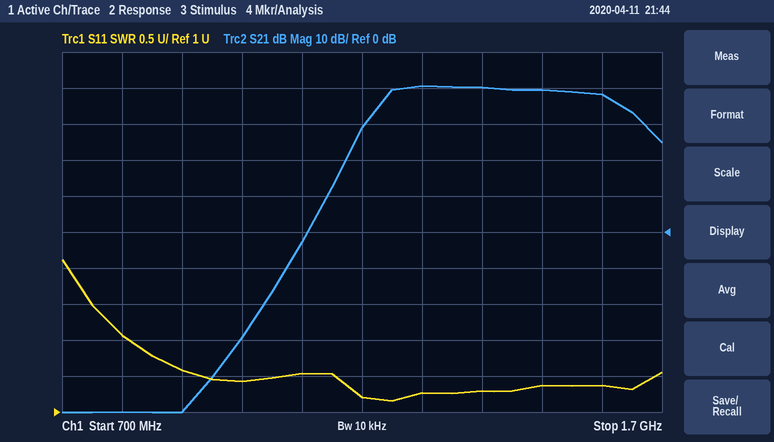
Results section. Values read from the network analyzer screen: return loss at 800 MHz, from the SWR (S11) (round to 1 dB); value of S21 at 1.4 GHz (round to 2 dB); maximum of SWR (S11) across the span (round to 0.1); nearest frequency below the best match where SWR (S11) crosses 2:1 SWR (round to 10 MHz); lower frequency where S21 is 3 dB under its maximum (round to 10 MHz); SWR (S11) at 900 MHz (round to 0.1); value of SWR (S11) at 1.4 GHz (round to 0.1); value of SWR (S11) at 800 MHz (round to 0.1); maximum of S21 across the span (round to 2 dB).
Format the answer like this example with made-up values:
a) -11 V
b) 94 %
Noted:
a) 9 dB
b) 40 dB
c) 3.1
d) 810 MHz
e) 1.24 GHz
f) 1.6
g) 1.3
h) 2.1
i) 40 dB
